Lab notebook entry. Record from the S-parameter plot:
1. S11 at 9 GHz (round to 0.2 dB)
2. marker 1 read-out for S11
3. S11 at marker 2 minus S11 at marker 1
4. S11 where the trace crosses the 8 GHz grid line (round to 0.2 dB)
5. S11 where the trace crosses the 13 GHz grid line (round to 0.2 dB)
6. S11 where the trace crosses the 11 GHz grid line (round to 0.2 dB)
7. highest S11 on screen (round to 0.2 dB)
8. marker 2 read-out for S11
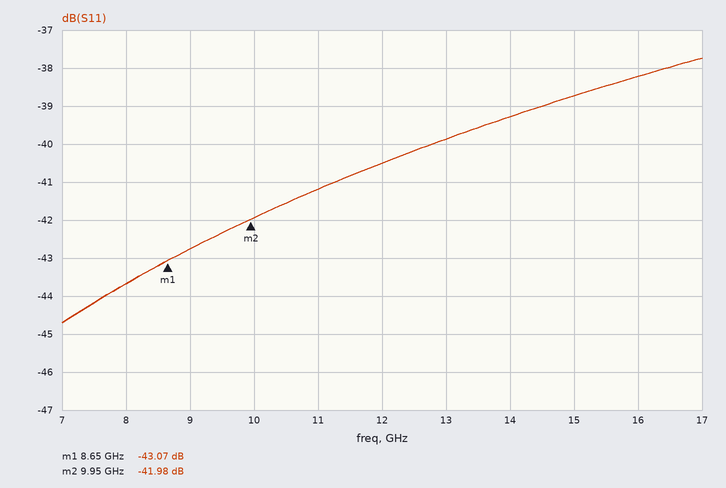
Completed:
-42.8 dB
-43.07 dB
1.09 dB
-43.6 dB
-39.8 dB
-41.2 dB
-37.8 dB
-41.98 dB
